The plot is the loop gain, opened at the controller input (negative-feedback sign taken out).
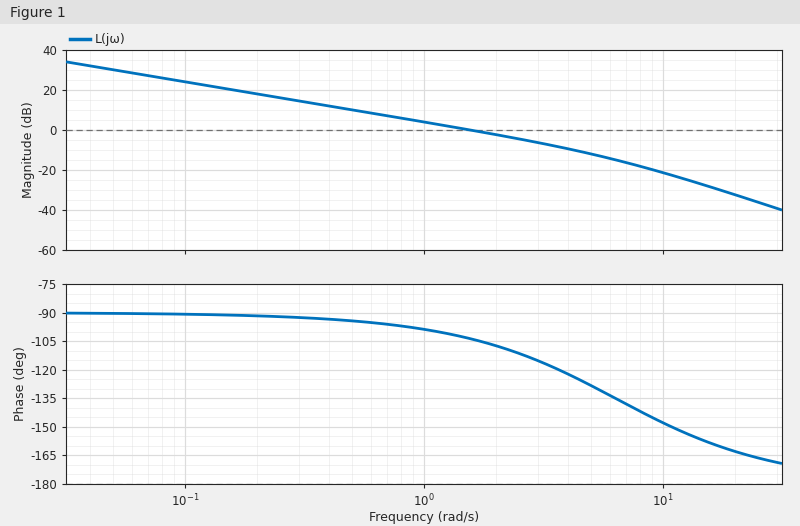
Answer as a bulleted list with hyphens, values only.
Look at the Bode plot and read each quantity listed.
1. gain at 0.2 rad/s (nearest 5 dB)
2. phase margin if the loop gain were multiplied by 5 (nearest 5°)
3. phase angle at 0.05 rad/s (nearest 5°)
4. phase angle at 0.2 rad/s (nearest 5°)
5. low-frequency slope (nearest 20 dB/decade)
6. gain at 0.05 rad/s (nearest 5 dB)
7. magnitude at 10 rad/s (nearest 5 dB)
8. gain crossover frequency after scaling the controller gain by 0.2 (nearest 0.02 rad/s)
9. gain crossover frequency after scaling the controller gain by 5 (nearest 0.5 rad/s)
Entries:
- 20 dB
- 45°
- -90°
- -90°
- -20 dB/decade
- 30 dB
- -20 dB
- 0.32 rad/s
- 6.0 rad/s
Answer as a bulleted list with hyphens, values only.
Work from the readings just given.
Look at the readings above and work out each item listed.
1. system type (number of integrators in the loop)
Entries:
- 1
